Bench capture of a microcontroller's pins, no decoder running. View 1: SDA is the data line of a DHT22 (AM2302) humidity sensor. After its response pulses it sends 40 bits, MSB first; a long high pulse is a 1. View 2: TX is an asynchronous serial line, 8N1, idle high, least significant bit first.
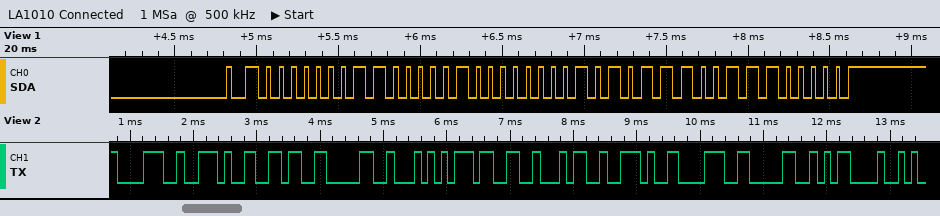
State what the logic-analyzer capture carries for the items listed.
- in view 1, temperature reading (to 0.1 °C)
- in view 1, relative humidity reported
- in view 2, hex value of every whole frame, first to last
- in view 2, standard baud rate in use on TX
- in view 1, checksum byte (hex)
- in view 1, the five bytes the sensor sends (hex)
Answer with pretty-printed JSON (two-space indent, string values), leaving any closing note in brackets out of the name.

{
  "in view 1, temperature reading": "34.8 °C",
  "in view 1, relative humidity reported": "38.6 %",
  "in view 2, hex value of every whole frame, first to last": "38 2E 36 30 54 33 34 2E 38 30 0D",
  "in view 2, standard baud rate in use on TX": "9600 baud",
  "in view 1, checksum byte": "0xE0",
  "in view 1, the five bytes the sensor sends": "01 82 01 5C E0"
}
